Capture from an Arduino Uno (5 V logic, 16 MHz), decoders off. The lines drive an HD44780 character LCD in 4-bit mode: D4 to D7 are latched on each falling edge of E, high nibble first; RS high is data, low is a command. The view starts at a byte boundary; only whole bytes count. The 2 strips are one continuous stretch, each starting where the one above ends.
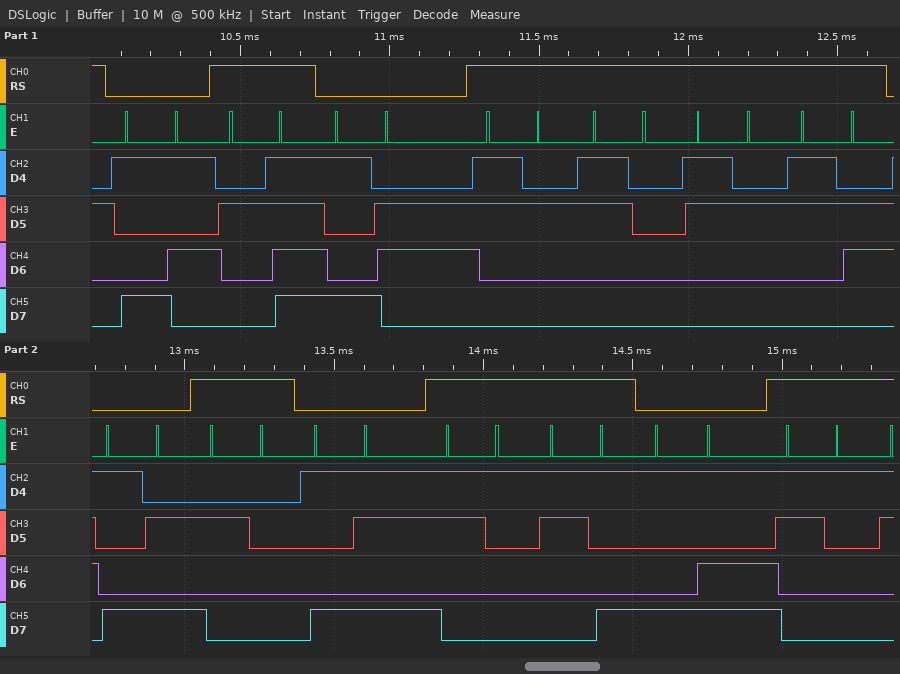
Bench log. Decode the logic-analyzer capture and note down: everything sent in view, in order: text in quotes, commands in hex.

0x95 "/" 0x96 "2026" 0x9A " " 0x9B "19" 0x9D "1"
